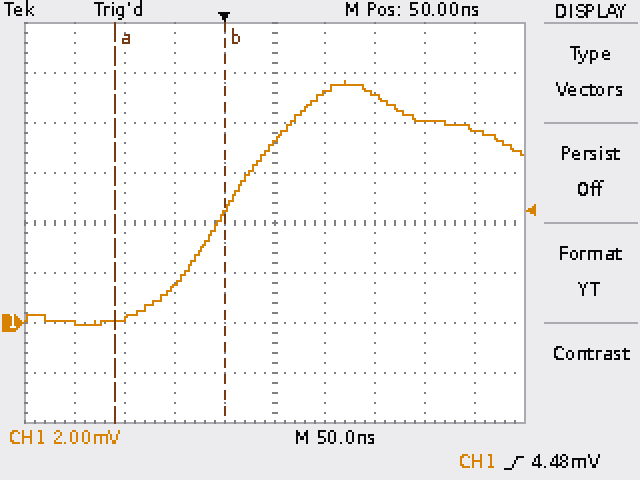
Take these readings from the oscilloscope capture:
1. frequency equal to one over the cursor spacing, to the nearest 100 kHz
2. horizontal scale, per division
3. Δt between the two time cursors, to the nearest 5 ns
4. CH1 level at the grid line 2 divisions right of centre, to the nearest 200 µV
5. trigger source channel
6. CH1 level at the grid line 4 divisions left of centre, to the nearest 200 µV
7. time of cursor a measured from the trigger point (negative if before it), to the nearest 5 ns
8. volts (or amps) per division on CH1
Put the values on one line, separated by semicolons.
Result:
9.1 MHz; 50 ns; 110 ns; 9.2 mV; CH1; 0.0 mV; -110 ns; 2 mV
